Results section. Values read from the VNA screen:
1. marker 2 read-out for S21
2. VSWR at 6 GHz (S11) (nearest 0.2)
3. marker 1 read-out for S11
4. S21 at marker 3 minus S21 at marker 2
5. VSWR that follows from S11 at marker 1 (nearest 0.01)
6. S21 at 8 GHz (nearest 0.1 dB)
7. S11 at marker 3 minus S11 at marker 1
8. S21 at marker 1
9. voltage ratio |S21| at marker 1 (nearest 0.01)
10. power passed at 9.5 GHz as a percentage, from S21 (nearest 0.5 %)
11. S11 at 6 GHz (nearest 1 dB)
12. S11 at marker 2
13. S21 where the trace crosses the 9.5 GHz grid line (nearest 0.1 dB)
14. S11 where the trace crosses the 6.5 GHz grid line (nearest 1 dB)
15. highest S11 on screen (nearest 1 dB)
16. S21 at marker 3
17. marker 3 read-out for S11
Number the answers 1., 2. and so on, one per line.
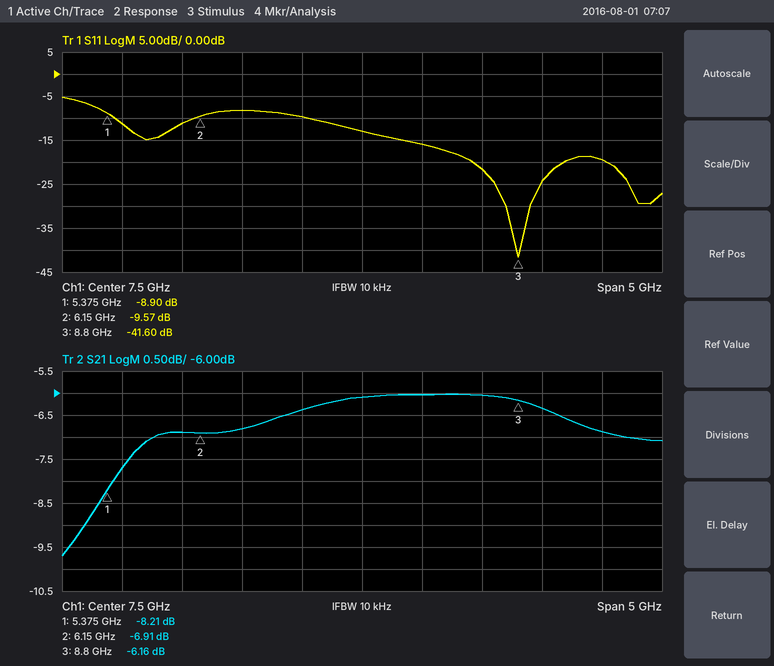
1. -6.91 dB
2. 1.8
3. -8.90 dB
4. 0.75 dB
5. 2.12
6. -6.0 dB
7. -32.70 dB
8. -8.21 dB
9. 0.39
10. 20.5 %
11. -11 dB
12. -9.57 dB
13. -6.9 dB
14. -8 dB
15. -5 dB
16. -6.16 dB
17. -41.60 dB
